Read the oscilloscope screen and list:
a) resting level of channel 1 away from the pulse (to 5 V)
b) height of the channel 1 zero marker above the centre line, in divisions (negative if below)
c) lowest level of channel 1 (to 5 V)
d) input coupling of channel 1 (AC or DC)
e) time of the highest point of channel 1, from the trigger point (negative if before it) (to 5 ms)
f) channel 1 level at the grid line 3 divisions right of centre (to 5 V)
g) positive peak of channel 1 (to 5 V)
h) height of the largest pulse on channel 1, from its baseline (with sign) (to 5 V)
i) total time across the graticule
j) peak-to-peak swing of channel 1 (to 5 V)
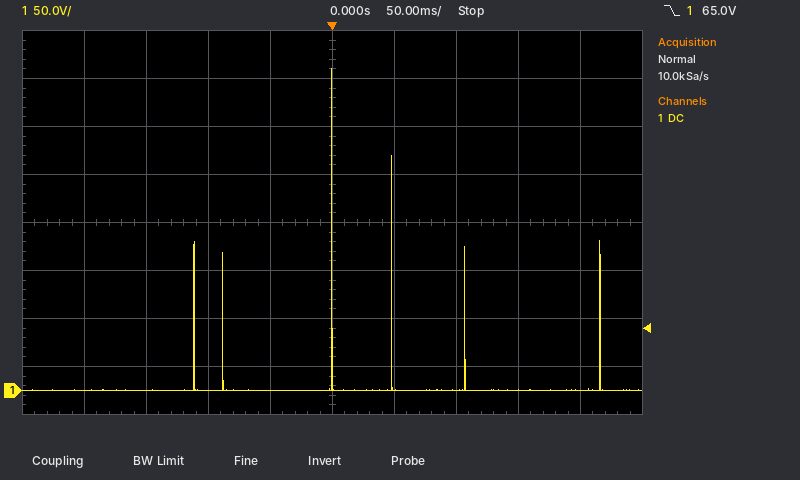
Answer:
0 V
-3.5 div
0 V
DC
0 ms
0 V
335 V
+335 V
500 ms
335 V
